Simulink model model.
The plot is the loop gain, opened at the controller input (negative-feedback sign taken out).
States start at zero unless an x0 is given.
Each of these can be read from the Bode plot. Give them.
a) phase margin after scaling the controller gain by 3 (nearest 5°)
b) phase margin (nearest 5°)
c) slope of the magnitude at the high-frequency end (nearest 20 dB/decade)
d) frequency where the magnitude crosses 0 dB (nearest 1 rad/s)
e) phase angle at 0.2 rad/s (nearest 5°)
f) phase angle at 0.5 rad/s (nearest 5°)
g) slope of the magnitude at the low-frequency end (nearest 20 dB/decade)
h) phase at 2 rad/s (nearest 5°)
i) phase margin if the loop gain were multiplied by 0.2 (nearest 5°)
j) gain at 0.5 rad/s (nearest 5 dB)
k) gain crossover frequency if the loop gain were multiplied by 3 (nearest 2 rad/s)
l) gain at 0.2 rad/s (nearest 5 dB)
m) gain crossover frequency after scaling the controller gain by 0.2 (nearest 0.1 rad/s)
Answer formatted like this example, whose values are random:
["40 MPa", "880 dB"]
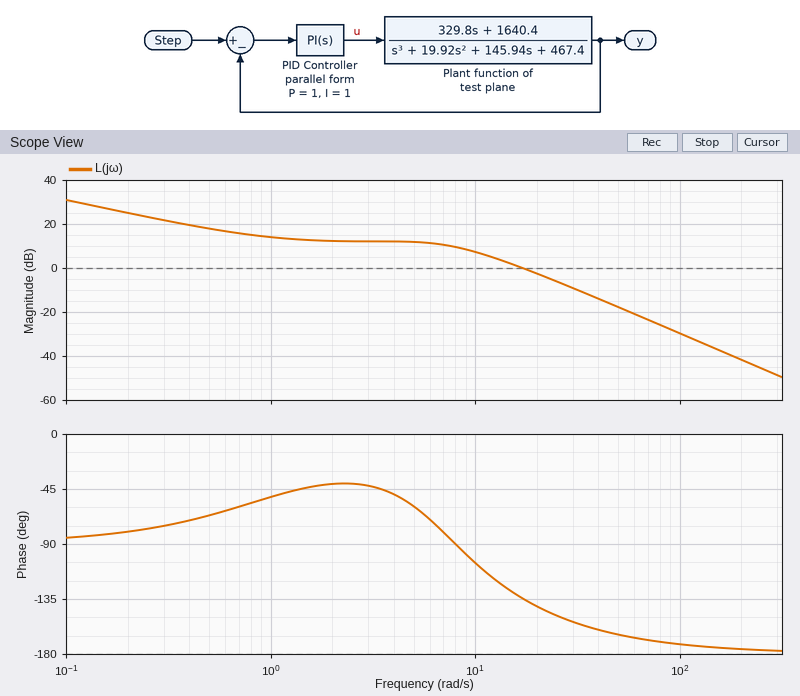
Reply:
["25°", "45°", "-40 dB/decade", "17 rad/s", "-80°", "-65°", "-20 dB/decade", "-40°", "130°", "20 dB", "30 rad/s", "25 dB", "1.0 rad/s"]
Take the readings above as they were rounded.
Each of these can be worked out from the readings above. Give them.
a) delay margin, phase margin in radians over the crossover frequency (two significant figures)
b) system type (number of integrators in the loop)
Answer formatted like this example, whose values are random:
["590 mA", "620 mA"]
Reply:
["0.046 s", "1"]
